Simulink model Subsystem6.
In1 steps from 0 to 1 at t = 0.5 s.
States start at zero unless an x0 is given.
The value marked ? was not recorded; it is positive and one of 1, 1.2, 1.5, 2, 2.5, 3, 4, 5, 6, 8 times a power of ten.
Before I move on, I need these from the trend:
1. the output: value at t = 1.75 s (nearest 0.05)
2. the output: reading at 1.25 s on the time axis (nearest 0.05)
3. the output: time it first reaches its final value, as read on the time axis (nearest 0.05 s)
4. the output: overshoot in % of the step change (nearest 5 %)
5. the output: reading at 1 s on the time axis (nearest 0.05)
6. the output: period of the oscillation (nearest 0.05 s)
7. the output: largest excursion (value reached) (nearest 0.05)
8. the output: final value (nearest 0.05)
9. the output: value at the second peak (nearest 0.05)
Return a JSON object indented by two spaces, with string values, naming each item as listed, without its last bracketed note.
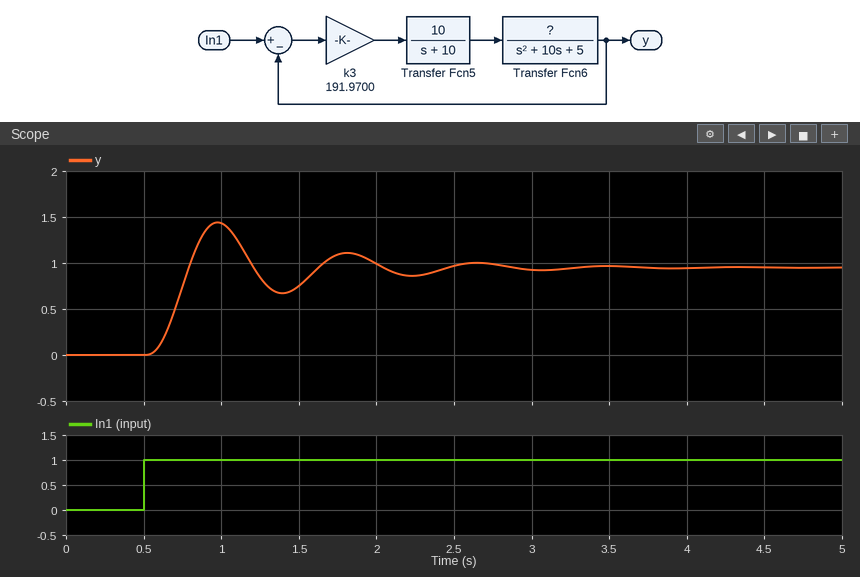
{
  "the output: value at t = 1.75 s": "1.10",
  "the output: reading at 1.25 s on the time axis": "0.85",
  "the output: time it first reaches its final value, as read on the time axis": "0.80 s",
  "the output: overshoot in % of the step change": "50 %",
  "the output: reading at 1 s on the time axis": "1.45",
  "the output: period of the oscillation": "0.85 s",
  "the output: largest excursion (value reached)": "1.45",
  "the output: final value": "0.95",
  "the output: value at the second peak": "1.10"
}
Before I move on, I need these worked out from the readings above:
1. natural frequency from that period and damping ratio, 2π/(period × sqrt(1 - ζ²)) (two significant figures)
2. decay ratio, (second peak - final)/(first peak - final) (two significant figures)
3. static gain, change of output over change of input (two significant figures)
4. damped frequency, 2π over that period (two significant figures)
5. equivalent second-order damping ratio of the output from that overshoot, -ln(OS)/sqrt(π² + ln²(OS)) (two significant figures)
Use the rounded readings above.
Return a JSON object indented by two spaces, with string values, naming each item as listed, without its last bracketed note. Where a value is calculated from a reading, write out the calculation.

{
  "natural frequency from that period and damping ratio, 2π/(period × sqrt(1 - ζ²))": "2π / (0.85 × sqrt(1 - 0.22²)) = 7.6 rad/s",
  "decay ratio, (second peak - final)/(first peak - final)": "(1.1 - 0.95) / (1.45 - 0.95) = 0.30",
  "static gain, change of output over change of input": "(0.95 - 0) / (1 - 0) = 0.95",
  "damped frequency, 2π over that period": "2π / 0.85 = 7.4 rad/s",
  "equivalent second-order damping ratio of the output from that overshoot, -ln(OS)/sqrt(π² + ln²(OS))": "ln(0.5) = -0.693; 0.693 / sqrt(9.870 + 0.480) = 0.22"
}
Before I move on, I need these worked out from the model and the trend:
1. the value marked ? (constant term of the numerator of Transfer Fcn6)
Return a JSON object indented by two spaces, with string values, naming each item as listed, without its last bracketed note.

{
  "the value marked ?": "0.5"
}
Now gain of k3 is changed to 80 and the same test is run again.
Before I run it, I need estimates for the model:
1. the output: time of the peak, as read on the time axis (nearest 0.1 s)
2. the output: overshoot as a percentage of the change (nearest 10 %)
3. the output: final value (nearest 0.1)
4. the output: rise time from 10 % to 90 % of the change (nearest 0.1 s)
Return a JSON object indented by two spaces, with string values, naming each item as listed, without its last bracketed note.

{
  "the output: time of the peak, as read on the time axis": "1.2 s",
  "the output: overshoot as a percentage of the change": "20 %",
  "the output: final value": "0.9",
  "the output: rise time from 10 % to 90 % of the change": "0.3 s"
}
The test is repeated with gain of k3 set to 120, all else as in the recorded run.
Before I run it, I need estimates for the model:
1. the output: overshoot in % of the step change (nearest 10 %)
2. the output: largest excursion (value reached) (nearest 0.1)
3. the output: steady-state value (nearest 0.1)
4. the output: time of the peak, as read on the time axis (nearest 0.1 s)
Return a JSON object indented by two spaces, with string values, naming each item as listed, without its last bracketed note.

{
  "the output: overshoot in % of the step change": "30 %",
  "the output: largest excursion (value reached)": "1.2",
  "the output: steady-state value": "0.9",
  "the output: time of the peak, as read on the time axis": "1.1 s"
}
